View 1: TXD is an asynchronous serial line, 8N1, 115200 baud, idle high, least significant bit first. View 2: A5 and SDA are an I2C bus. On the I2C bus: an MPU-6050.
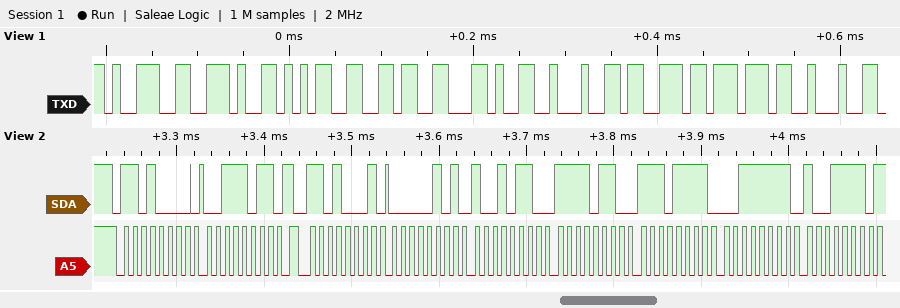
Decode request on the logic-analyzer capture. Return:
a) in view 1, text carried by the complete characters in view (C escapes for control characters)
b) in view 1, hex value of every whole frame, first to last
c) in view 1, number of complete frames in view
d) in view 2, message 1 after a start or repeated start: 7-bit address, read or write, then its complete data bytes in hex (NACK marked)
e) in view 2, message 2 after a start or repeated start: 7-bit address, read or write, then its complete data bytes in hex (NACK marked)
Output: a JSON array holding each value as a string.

["\"9.56,\\\"sw\\\"\"", "39 2E 35 36 2C 22 73 77 22", "9", "0x68 write: 3B", "0x68 read: 05 96 F6 EF 3F 9E NACK"]
